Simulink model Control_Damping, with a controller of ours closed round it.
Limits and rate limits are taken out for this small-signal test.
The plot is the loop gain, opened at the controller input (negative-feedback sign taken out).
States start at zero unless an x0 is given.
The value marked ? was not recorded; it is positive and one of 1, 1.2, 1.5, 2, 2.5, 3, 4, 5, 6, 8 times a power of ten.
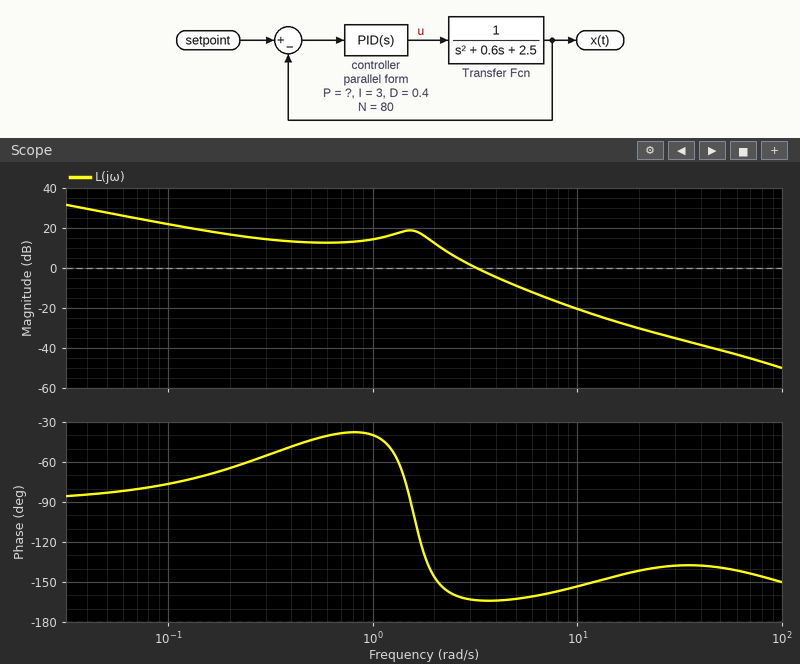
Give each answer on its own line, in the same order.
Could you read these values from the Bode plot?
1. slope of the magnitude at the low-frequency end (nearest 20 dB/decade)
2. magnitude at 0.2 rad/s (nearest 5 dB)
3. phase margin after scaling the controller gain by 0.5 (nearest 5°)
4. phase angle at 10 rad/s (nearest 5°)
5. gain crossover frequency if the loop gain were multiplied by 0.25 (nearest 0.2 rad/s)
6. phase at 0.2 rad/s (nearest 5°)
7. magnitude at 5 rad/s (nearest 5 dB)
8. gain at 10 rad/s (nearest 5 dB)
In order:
-20 dB/decade
15 dB
20°
-155°
2.0 rad/s
-65°
-10 dB
-20 dB
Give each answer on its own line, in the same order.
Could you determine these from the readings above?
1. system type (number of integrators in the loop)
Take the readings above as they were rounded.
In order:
1
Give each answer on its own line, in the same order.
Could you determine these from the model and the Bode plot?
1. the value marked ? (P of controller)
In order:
8
